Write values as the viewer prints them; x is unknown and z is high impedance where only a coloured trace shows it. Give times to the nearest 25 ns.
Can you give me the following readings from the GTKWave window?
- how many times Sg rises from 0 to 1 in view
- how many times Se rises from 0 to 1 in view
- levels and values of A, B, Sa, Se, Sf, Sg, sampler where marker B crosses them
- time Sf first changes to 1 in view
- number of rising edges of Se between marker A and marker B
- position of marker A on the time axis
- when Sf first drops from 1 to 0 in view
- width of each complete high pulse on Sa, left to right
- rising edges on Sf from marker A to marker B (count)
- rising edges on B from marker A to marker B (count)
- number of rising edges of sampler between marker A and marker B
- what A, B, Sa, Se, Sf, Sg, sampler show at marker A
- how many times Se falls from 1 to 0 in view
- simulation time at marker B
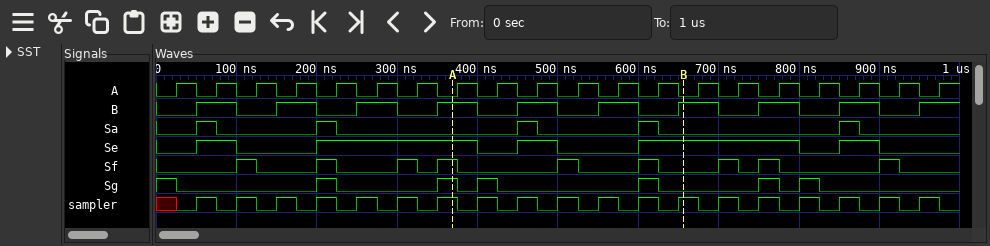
6
5
A=0, B=1, Sa=0, Se=1, Sf=0, Sg=0, sampler=1
100 ns
2
375 ns
125 ns
25 ns, 25 ns, 25 ns, 25 ns, 25 ns
2
3
6
A=0, B=1, Sa=0, Se=1, Sf=1, Sg=1, sampler=1
5
650 ns
